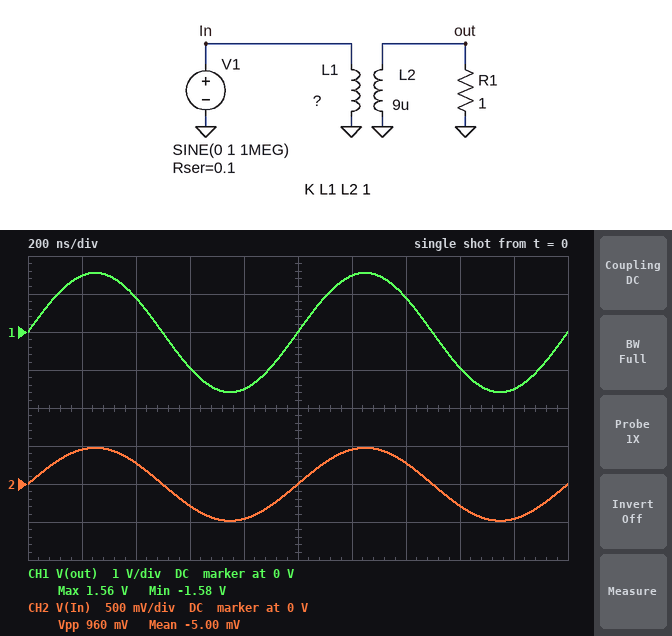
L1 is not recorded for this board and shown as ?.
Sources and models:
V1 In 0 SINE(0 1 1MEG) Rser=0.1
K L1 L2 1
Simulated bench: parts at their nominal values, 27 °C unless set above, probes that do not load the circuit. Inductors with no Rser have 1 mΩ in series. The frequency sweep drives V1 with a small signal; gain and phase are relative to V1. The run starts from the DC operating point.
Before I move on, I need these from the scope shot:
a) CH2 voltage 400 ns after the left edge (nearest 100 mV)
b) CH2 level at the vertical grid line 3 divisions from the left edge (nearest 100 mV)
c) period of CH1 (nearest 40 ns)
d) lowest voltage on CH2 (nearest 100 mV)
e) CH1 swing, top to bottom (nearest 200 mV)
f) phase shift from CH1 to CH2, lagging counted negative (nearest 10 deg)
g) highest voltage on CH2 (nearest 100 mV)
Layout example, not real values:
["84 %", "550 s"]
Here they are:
["300 mV", "-300 mV", "1.00 µs", "-500 mV", "3.2 V", "0 deg", "500 mV"]
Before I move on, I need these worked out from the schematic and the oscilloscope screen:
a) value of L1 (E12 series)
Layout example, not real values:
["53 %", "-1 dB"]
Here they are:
["820 nH"]
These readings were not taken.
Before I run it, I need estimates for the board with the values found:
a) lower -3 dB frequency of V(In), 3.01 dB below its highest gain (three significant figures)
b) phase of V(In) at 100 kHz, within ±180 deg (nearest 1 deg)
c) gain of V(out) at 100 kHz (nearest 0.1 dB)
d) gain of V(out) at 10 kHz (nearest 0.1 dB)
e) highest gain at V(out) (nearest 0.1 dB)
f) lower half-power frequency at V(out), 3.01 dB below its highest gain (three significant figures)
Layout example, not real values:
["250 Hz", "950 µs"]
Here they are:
["9.30 kHz", "5 deg", "3.9 dB", "1.2 dB", "3.9 dB", "9.30 kHz"]
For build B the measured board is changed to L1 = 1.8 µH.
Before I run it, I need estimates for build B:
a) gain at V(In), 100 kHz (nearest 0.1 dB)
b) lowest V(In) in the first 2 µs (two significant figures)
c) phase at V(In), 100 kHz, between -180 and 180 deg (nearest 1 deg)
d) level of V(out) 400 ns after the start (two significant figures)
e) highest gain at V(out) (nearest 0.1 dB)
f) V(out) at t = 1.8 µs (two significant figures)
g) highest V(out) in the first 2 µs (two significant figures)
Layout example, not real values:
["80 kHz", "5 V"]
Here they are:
["-3.5 dB", "-670 mV", "3 deg", "860 mV", "3.4 dB", "-1.4 V", "1.5 V"]
